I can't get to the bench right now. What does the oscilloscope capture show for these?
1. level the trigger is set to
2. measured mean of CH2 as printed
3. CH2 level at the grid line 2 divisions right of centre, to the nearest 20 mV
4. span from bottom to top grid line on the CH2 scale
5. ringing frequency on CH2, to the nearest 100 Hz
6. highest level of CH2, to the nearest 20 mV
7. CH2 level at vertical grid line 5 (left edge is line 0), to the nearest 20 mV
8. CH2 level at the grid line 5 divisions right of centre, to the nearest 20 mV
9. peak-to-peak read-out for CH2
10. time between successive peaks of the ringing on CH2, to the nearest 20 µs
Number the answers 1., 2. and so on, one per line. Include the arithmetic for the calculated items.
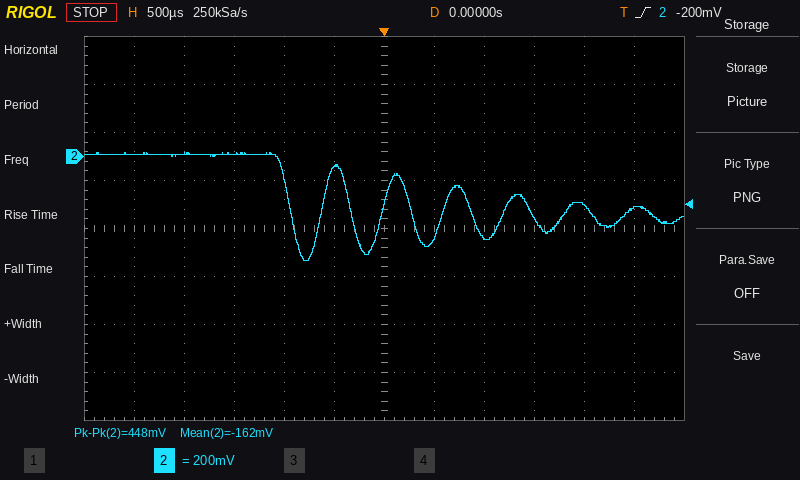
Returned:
1. -200 mV
2. -162 mV
3. -340 mV
4. 1.6 V
5. 1 / 600 µs ≈ 1.7 kHz
6. 20 mV
7. -40 mV
8. -220 mV
9. 448 mV
10. 600 µs
